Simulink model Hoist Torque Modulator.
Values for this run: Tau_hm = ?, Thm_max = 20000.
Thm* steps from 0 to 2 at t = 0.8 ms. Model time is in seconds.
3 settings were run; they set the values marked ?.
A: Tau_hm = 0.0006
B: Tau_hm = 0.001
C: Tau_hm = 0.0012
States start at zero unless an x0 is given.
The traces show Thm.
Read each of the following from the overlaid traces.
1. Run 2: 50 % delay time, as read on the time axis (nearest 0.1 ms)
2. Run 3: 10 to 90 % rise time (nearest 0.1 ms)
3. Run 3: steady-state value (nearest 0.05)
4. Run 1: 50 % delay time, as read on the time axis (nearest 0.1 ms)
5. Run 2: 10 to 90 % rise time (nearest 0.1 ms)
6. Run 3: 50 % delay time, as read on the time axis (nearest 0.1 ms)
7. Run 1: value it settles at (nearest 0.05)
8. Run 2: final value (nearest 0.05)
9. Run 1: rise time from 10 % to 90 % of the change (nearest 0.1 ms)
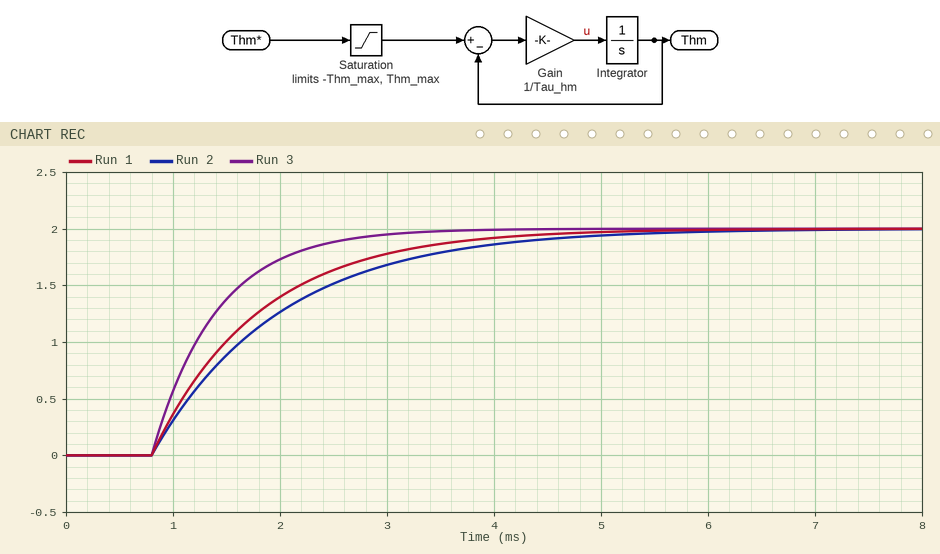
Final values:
1.6 ms
1.3 ms
2.00
1.5 ms
2.6 ms
1.2 ms
2.00
2.00
2.2 ms
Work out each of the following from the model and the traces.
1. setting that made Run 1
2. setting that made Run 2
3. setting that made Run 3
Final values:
B
C
A
